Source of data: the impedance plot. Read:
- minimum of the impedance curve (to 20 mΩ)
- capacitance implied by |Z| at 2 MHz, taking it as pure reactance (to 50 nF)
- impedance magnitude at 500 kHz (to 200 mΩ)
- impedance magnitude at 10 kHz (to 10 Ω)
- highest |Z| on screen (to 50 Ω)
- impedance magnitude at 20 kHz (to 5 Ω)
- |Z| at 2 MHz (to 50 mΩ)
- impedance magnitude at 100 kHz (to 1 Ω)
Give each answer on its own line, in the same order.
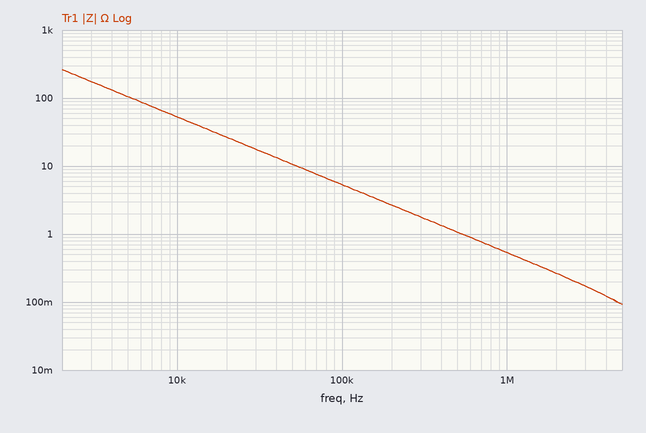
100 mΩ
300 nF
1.0 Ω
50 Ω
250 Ω
25 Ω
250 mΩ
5 Ω
